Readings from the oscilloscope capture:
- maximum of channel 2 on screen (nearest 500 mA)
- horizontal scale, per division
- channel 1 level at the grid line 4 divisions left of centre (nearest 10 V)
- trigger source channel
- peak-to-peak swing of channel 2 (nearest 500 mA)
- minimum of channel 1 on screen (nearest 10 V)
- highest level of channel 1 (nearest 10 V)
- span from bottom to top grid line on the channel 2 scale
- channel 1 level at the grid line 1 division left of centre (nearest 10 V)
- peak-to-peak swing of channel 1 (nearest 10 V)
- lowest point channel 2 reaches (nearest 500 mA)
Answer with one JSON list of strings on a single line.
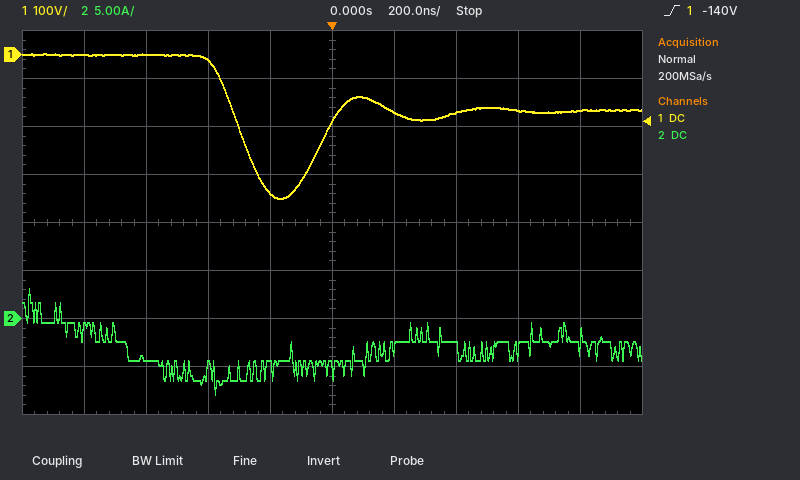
["3.0 A", "200 ns", "0 V", "channel 1", "11.0 A", "-300 V", "0 V", "40 A", "-290 V", "300 V", "-8.0 A"]
